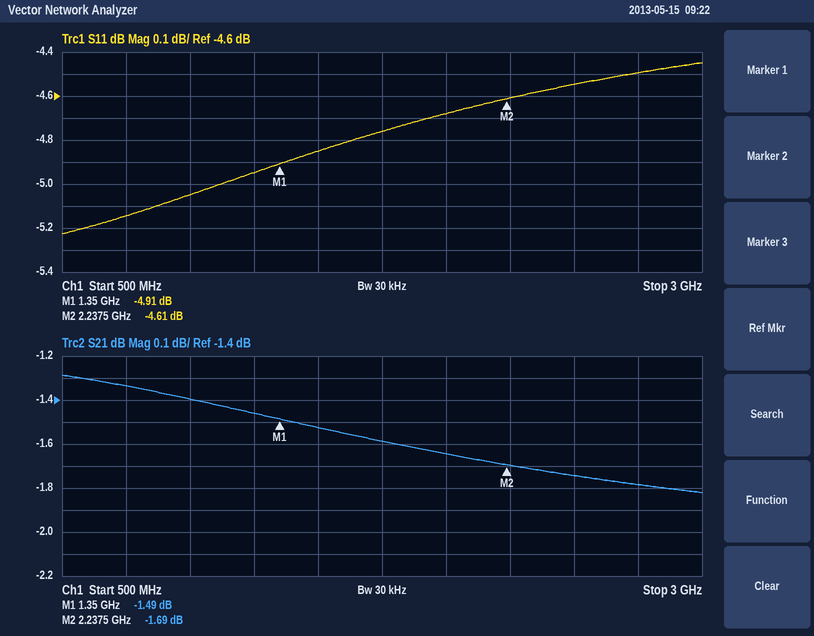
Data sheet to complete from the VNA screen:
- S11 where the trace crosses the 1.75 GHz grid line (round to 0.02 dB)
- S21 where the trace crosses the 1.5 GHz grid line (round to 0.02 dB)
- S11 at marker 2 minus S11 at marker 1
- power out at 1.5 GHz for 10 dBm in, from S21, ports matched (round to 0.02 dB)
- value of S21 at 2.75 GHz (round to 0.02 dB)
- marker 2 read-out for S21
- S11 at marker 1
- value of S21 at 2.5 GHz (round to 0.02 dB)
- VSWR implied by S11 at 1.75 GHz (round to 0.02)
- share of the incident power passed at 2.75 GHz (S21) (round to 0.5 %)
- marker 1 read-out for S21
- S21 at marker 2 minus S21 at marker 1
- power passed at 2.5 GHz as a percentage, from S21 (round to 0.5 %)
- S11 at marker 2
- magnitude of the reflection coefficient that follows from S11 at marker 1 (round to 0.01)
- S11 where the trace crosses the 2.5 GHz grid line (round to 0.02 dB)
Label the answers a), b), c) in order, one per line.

a) -4.76 dB
b) -1.52 dB
c) 0.30 dB
d) 8.48 dBm
e) -1.78 dB
f) -1.69 dB
g) -4.91 dB
h) -1.74 dB
i) 3.74
j) 66.5 %
k) -1.49 dB
l) -0.20 dB
m) 67.0 %
n) -4.61 dB
o) 0.57
p) -4.54 dB
